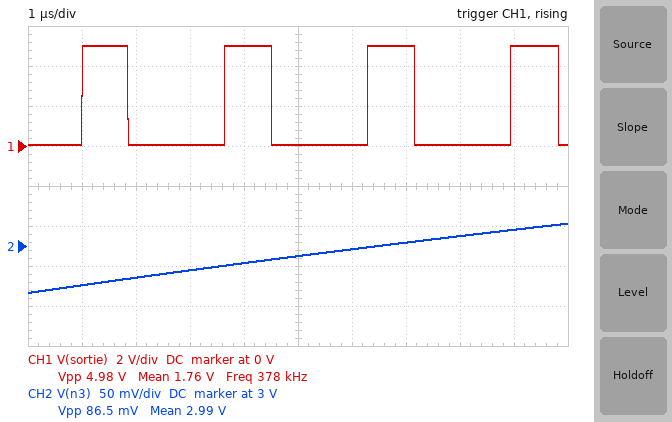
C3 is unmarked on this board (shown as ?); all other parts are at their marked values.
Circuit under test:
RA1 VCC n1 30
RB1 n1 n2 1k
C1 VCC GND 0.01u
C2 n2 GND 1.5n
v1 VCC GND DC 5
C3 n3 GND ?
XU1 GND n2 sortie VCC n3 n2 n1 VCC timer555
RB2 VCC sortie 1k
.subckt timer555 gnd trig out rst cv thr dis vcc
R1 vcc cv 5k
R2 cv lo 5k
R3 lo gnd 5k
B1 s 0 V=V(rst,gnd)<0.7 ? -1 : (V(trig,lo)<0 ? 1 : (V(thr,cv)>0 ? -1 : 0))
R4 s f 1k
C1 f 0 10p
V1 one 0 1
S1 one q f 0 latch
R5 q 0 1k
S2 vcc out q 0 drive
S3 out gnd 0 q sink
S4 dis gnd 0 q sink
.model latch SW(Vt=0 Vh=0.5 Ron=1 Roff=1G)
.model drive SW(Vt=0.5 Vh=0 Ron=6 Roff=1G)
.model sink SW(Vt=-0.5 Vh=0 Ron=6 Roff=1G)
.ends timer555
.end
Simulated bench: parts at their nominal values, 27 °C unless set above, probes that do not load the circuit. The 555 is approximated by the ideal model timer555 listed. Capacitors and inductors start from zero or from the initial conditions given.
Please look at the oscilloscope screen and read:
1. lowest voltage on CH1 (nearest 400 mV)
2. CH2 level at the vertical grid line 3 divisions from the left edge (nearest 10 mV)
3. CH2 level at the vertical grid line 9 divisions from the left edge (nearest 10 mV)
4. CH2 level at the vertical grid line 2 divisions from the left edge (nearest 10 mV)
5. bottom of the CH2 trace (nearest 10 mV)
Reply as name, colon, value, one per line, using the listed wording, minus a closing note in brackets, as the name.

lowest voltage on CH1: 0 V
CH2 level at the vertical grid line 3 divisions from the left edge: 2.97 V
CH2 level at the vertical grid line 9 divisions from the left edge: 3.02 V
CH2 level at the vertical grid line 2 divisions from the left edge: 2.96 V
bottom of the CH2 trace: 2.94 V
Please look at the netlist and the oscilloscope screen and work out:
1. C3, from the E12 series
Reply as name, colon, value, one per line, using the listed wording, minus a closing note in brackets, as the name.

C3, from the E12 series: 12 nF
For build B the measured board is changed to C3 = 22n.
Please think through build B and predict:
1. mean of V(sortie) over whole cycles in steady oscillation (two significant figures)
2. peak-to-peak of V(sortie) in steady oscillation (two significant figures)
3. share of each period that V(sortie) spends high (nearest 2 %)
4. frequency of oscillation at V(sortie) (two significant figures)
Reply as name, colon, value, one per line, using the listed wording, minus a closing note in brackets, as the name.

mean of V(sortie) over whole cycles in steady oscillation: 1.1 V
peak-to-peak of V(sortie) in steady oscillation: 5.0 V
share of each period that V(sortie) spends high: 22 %
frequency of oscillation at V(sortie): 370 kHz
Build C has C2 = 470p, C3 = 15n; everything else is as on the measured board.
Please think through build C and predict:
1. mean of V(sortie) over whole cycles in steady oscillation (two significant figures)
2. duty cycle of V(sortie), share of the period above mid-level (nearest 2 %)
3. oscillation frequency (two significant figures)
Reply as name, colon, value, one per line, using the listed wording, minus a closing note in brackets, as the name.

mean of V(sortie) over whole cycles in steady oscillation: 1.5 V
duty cycle of V(sortie), share of the period above mid-level: 30 %
oscillation frequency: 1.2 MHz
